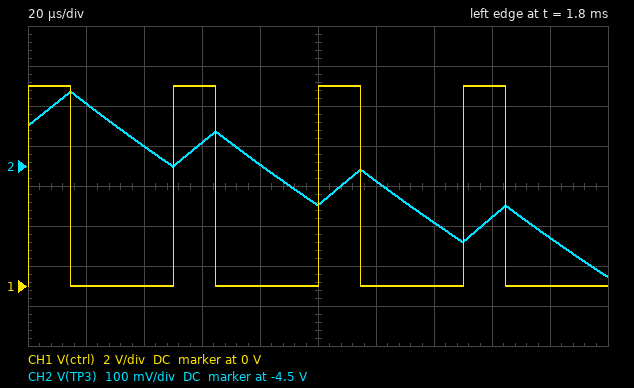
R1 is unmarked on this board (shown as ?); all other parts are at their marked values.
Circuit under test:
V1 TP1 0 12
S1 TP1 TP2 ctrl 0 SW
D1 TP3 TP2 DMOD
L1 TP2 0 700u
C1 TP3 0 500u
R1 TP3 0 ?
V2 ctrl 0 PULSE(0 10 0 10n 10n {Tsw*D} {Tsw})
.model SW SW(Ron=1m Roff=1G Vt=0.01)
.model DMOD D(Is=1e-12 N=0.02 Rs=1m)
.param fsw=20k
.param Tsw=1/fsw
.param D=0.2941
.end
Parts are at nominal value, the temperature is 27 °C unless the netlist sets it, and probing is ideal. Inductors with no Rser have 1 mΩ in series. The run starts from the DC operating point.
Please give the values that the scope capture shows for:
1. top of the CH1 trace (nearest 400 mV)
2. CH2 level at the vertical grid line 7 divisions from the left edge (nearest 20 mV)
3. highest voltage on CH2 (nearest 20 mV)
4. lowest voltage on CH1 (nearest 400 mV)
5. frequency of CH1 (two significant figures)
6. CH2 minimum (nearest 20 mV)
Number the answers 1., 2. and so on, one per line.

1. 10.0 V
2. -4.64 V
3. -4.32 V
4. 0 V
5. 20 kHz
6. -4.78 V
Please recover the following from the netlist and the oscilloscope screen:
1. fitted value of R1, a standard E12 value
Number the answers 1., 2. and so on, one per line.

1. 1.5 Ω
